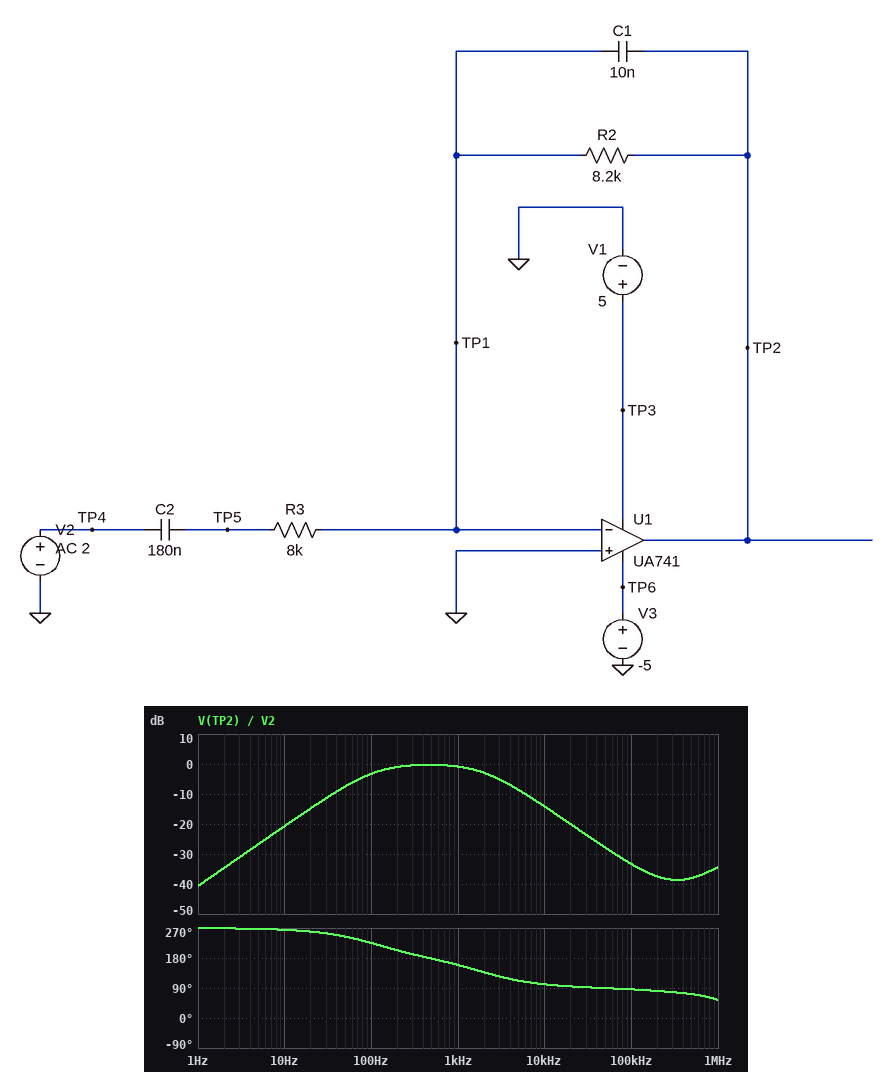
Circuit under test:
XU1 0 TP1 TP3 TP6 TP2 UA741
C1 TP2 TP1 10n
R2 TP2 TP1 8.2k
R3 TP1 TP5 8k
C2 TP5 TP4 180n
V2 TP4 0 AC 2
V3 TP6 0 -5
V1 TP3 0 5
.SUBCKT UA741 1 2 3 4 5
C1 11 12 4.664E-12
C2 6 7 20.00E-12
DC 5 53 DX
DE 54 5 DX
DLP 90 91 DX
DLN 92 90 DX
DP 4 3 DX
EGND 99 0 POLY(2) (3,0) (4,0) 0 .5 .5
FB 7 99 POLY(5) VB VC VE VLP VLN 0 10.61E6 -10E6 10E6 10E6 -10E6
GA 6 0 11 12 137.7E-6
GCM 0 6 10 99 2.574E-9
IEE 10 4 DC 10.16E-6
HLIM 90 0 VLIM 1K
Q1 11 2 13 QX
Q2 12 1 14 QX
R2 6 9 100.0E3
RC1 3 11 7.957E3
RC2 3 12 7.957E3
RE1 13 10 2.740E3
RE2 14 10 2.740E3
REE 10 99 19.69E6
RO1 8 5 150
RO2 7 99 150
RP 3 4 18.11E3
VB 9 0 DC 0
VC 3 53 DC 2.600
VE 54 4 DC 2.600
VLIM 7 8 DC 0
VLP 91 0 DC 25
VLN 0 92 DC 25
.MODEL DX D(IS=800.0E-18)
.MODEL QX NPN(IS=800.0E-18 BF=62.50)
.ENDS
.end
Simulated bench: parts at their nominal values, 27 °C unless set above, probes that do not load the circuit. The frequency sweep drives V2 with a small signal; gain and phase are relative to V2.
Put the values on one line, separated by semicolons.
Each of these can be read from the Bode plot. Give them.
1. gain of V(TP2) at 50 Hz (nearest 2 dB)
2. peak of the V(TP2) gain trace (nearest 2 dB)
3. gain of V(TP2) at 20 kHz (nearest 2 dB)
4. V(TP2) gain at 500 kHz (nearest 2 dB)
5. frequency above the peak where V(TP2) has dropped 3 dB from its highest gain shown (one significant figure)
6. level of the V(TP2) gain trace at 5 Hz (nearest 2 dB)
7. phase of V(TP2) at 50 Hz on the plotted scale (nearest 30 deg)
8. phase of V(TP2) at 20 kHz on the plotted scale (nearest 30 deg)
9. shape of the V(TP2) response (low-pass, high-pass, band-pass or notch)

-8 dB; 0 dB; -20 dB; -38 dB; 2 kHz; -26 dB; 240 deg; 90 deg; band-pass
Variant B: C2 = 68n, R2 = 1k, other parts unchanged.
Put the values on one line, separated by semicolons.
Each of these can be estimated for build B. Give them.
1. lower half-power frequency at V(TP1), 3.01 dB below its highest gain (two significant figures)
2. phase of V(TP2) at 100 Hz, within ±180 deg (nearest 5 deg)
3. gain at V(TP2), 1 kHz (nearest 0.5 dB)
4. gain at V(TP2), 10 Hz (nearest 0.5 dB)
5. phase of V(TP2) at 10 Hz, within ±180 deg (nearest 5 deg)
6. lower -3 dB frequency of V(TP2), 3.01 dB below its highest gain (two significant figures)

940 kHz; -110 deg; -18.5 dB; -47.5 dB; -90 deg; 280 Hz
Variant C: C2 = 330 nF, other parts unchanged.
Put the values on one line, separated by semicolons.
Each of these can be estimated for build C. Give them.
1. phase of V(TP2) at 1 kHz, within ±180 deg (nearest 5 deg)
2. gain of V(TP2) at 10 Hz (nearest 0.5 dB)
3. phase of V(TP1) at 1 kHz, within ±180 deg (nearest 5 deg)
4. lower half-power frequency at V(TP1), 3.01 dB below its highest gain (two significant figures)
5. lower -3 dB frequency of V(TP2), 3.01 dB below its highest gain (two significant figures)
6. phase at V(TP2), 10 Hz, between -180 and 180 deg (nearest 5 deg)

155 deg; -15.5 dB; 65 deg; 940 kHz; 57 Hz; -100 deg
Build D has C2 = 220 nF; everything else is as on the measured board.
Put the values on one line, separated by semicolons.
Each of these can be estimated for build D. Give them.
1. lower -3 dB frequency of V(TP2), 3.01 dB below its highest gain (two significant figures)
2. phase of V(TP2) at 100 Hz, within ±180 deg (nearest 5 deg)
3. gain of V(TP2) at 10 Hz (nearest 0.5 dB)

83 Hz; -140 deg; -19.0 dB
